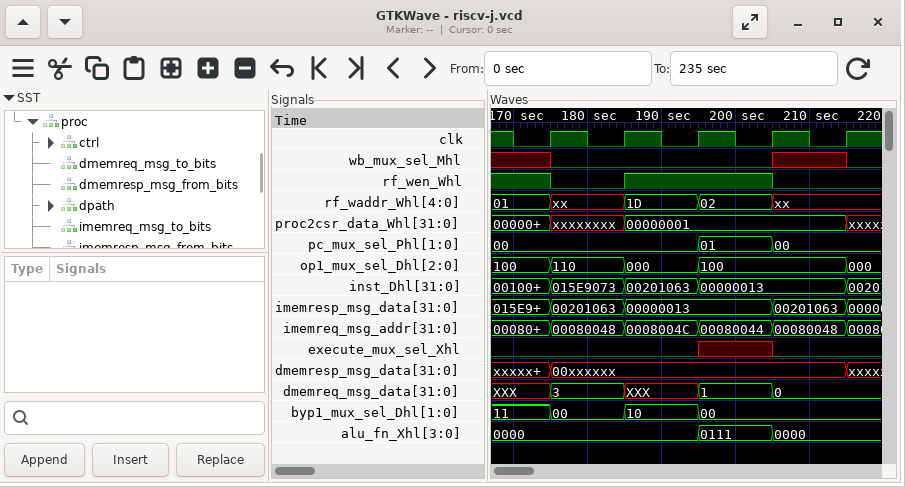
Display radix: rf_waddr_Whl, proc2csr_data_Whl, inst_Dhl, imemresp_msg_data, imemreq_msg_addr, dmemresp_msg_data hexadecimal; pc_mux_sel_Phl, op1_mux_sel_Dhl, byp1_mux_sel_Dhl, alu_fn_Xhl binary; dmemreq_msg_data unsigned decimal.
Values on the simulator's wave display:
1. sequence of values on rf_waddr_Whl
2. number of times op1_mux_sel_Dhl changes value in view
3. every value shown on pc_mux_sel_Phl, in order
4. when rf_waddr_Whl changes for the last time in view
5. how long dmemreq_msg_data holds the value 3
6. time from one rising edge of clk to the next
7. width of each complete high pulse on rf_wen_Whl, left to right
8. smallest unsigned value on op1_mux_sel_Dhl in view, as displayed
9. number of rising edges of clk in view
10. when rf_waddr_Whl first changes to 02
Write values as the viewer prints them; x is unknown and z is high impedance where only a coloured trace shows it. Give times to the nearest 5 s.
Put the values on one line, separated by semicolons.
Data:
01, xx, 1D, 02, xx; 4; 00, 01, 00; 205 s; 10 s; 10 s; 20 s; 000; 5; 195 s
